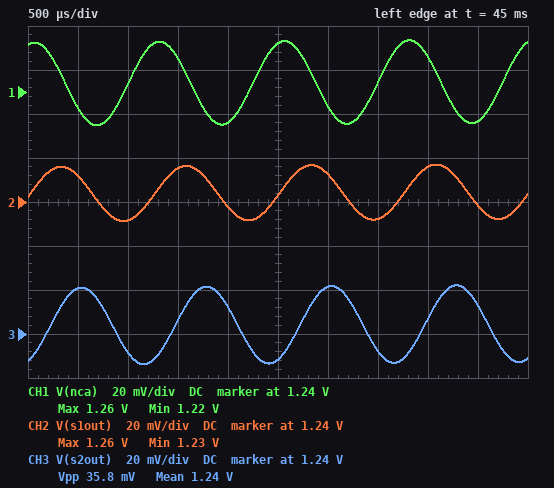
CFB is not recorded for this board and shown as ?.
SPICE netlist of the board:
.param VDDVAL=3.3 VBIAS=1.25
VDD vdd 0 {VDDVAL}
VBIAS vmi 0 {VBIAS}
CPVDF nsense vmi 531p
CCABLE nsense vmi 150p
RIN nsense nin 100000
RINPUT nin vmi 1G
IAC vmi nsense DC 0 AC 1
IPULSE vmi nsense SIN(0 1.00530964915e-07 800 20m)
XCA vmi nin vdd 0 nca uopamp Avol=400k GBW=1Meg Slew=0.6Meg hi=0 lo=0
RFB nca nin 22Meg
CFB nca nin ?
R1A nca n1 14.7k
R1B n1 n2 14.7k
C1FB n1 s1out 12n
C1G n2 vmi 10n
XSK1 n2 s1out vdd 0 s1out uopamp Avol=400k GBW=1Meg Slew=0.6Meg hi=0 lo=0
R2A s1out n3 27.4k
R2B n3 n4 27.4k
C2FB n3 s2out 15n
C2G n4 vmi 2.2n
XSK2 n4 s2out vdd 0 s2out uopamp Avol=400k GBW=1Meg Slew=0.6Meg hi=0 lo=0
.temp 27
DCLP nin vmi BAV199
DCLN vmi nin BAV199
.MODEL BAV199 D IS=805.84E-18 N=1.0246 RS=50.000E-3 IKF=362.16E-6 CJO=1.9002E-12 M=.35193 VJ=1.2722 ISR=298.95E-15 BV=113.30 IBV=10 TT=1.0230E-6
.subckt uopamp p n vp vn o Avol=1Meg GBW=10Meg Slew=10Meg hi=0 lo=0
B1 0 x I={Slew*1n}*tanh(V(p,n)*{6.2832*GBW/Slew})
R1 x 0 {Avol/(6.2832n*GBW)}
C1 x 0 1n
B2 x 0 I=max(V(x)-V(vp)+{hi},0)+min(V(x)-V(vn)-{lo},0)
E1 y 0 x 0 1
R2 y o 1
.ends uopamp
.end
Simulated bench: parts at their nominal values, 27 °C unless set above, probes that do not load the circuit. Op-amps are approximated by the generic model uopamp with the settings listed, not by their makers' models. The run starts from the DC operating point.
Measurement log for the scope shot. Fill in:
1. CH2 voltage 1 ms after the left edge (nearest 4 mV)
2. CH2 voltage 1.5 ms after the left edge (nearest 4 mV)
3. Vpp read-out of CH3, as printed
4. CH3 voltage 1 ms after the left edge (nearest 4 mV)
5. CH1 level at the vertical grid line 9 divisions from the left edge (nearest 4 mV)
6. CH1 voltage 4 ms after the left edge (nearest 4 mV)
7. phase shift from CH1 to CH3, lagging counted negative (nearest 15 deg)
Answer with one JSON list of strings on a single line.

["1.232 V", "1.256 V", "35.8 mV", "1.232 V", "1.228 V", "1.256 V", "-135 deg"]
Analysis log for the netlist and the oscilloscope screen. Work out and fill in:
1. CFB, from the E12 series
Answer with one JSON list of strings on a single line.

["1 nF"]
